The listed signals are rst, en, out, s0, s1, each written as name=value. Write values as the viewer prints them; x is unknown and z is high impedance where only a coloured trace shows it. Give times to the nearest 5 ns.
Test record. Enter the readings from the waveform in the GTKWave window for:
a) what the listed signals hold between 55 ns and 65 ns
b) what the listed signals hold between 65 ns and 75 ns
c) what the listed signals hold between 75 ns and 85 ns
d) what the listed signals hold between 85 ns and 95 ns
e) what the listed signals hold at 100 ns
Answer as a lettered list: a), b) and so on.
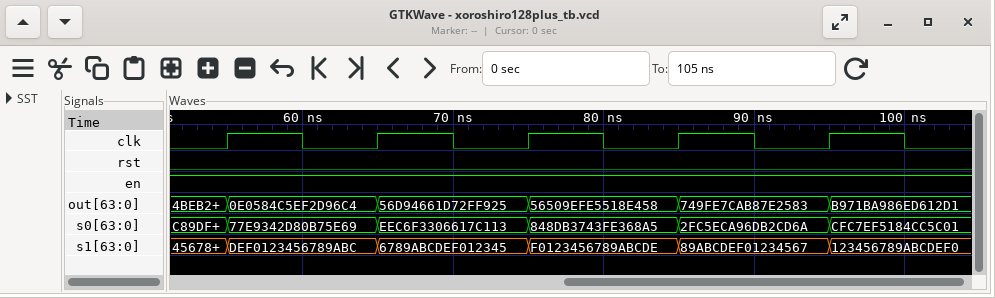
a) rst=0, en=1, out=0E0584C5EF2D96C4, s0=77E9342D80B75E69, s1=DEF0123456789ABC
b) rst=0, en=1, out=56D94661D72FF925, s0=EEC6F3306617C113, s1=6789ABCDEF012345
c) rst=0, en=1, out=56509EFE5518E458, s0=848DB3743FE368A5, s1=F0123456789ABCDE
d) rst=0, en=1, out=749FE7CAB87E2583, s0=2FC5ECA96DB2CD6A, s1=89ABCDEF01234567
e) rst=0, en=1, out=B971BA986ED612D1, s0=CFC7EF5184CC5C01, s1=123456789ABCDEF0
